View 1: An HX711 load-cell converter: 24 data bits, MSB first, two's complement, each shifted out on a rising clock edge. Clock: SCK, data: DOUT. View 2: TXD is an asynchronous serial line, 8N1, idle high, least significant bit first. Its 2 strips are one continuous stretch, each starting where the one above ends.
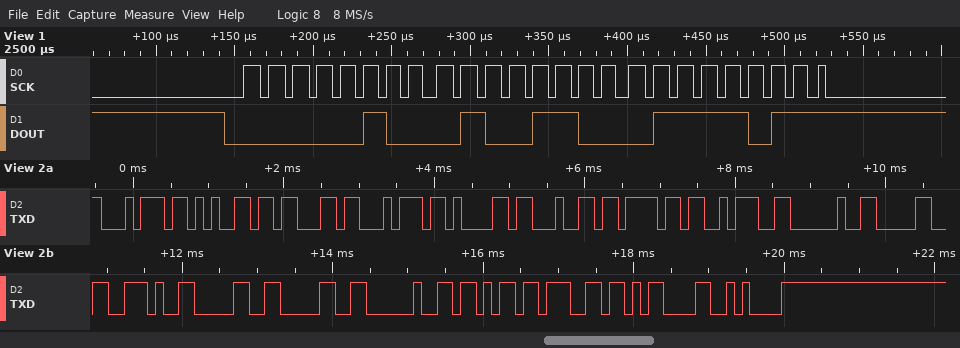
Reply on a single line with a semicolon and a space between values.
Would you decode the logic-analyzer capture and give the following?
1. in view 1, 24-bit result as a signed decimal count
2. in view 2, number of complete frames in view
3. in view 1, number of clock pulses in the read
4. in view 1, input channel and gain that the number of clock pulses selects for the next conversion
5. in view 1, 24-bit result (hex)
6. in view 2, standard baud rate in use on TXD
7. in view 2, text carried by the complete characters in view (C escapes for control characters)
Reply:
281723; 18; 25; channel A, gain 128; 0x044C7B; 9600 baud; "tectado: 0.00 kg\r\n"
